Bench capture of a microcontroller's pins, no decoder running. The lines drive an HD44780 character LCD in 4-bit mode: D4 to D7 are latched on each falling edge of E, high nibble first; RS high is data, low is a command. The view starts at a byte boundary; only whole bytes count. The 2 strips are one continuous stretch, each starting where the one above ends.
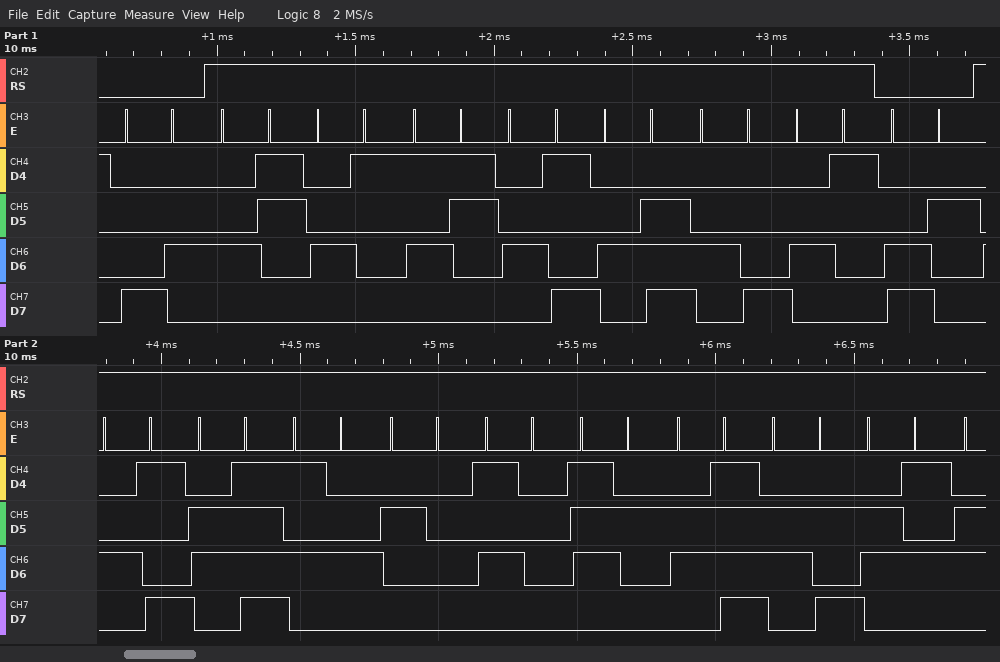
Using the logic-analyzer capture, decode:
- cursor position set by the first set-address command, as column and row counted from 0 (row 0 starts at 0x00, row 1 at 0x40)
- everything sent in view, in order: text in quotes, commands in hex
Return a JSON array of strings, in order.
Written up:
["column 4, row 0", "0x84 \"CASINHA\" 0xC2 \"IoT Proje\""]
